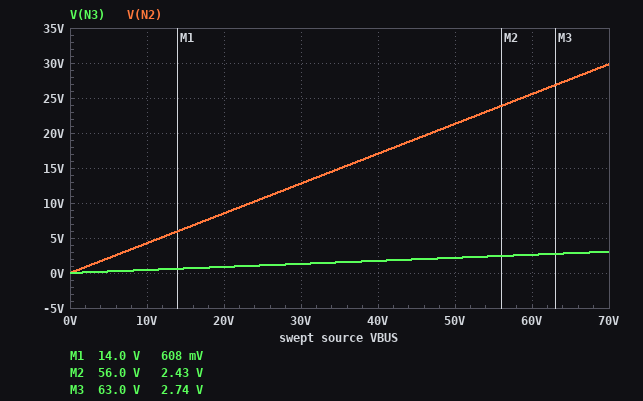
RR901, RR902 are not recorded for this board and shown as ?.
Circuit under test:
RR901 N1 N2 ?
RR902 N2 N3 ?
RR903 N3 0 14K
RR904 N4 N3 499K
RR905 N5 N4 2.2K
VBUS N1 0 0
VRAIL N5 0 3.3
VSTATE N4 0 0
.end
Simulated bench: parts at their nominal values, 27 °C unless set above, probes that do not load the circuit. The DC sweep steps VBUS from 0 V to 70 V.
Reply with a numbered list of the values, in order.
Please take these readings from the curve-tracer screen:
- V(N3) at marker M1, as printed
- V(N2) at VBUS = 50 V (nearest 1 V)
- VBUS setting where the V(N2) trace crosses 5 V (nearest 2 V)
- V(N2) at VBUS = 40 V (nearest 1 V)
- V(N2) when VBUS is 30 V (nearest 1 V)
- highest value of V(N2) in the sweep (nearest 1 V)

1. 608 mV
2. 21 V
3. 12 V
4. 17 V
5. 13 V
6. 30 V
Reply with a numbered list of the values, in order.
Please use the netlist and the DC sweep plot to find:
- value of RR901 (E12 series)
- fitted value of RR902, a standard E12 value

1. 180 kΩ
2. 120 kΩ
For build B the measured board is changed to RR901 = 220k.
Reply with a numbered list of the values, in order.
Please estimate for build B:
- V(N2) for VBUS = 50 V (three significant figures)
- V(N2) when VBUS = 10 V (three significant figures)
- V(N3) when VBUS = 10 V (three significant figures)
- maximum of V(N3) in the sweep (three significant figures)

1. 18.9 V
2. 3.78 V
3. 385 mV
4. 2.70 V
